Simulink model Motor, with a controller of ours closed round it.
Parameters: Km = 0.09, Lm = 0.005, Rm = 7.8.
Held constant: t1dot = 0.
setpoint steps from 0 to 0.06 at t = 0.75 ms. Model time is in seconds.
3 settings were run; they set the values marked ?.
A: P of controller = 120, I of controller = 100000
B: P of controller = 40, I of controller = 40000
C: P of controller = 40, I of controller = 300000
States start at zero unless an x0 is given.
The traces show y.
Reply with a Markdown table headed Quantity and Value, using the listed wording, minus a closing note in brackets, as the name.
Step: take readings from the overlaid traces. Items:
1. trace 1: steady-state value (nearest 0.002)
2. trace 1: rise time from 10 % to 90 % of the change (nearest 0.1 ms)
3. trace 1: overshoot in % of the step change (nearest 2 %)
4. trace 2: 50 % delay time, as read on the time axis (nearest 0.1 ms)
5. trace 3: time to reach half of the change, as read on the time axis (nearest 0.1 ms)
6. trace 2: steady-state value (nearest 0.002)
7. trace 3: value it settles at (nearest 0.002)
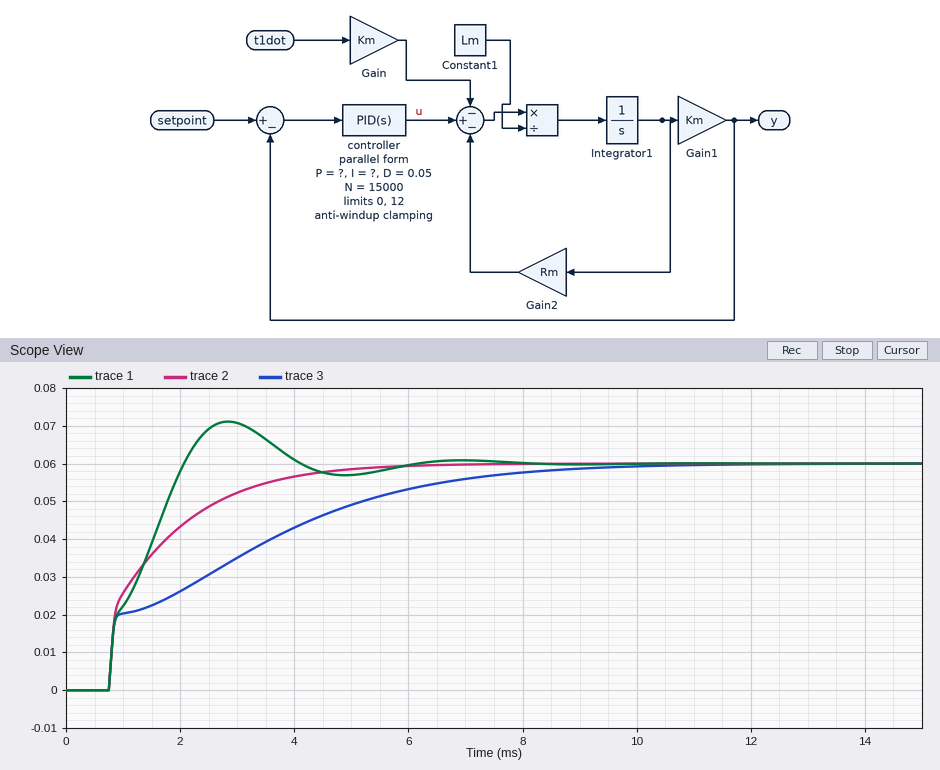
| Quantity | Value |
|---|---|
| trace 1: steady-state value | 0.060 |
| trace 1: rise time from 10 % to 90 % of the change | 1.1 ms |
| trace 1: overshoot in % of the step change | 18 % |
| trace 2: 50 % delay time, as read on the time axis | 1.2 ms |
| trace 3: time to reach half of the change, as read on the time axis | 2.4 ms |
| trace 2: steady-state value | 0.060 |
| trace 3: value it settles at | 0.060 |
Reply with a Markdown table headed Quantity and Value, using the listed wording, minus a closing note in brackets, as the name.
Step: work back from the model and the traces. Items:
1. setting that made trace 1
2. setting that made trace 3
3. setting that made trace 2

| Quantity | Value |
|---|---|
| setting that made trace 1 | C |
| setting that made trace 3 | B |
| setting that made trace 2 | A |
